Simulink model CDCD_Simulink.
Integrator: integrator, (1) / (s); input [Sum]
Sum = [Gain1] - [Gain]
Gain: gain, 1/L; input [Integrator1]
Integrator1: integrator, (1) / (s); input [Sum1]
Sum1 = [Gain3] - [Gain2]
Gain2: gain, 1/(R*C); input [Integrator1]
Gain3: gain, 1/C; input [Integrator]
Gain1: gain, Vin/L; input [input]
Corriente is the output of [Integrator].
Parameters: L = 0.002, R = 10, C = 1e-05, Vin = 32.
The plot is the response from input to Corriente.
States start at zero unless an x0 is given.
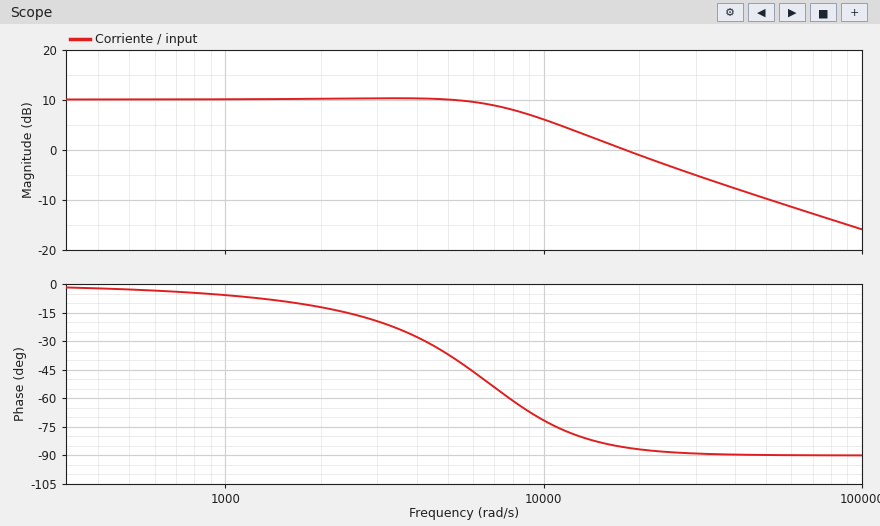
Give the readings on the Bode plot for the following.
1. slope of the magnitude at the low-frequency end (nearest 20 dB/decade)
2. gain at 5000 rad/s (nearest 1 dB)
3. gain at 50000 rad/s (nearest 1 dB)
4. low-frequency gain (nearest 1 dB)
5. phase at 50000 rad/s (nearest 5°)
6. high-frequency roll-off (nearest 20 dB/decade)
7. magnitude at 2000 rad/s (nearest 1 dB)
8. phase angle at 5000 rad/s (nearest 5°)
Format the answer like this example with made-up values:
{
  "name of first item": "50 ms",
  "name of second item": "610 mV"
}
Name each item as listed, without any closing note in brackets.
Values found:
{
  "slope of the magnitude at the low-frequency end": "0 dB/decade",
  "gain at 5000 rad/s": "10 dB",
  "gain at 50000 rad/s": "-10 dB",
  "low-frequency gain": "10 dB",
  "phase at 50000 rad/s": "-90°",
  "high-frequency roll-off": "-20 dB/decade",
  "magnitude at 2000 rad/s": "10 dB",
  "phase angle at 5000 rad/s": "-35°"
}
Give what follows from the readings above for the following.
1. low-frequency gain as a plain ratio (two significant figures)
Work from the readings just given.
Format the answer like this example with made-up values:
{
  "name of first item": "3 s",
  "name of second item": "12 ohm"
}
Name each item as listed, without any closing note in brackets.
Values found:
{
  "low-frequency gain as a plain ratio": "3.2"
}
